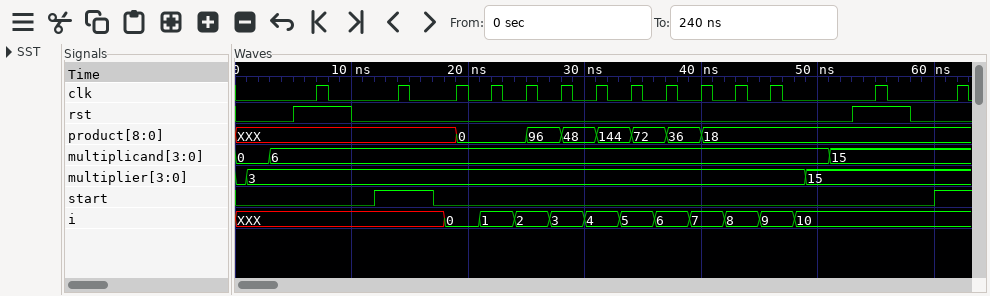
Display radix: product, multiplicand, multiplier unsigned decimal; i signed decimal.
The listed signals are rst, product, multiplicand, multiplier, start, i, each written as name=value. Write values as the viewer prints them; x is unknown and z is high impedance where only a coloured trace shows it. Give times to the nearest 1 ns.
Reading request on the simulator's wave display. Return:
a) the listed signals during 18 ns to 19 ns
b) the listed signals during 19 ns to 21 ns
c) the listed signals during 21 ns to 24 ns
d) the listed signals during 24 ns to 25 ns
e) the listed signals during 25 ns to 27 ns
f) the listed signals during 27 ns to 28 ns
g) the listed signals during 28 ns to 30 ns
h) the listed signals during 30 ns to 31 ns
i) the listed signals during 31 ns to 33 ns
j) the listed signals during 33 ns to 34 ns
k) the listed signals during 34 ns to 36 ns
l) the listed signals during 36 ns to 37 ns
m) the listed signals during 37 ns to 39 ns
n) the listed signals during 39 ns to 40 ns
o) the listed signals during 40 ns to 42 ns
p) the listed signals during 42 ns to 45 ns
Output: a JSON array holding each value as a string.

["rst=0, product=XXX, multiplicand=6, multiplier=3, start=0, i=0", "rst=0, product=0, multiplicand=6, multiplier=3, start=0, i=0", "rst=0, product=0, multiplicand=6, multiplier=3, start=0, i=1", "rst=0, product=0, multiplicand=6, multiplier=3, start=0, i=2", "rst=0, product=96, multiplicand=6, multiplier=3, start=0, i=2", "rst=0, product=96, multiplicand=6, multiplier=3, start=0, i=3", "rst=0, product=48, multiplicand=6, multiplier=3, start=0, i=3", "rst=0, product=48, multiplicand=6, multiplier=3, start=0, i=4", "rst=0, product=144, multiplicand=6, multiplier=3, start=0, i=4", "rst=0, product=144, multiplicand=6, multiplier=3, start=0, i=5", "rst=0, product=72, multiplicand=6, multiplier=3, start=0, i=5", "rst=0, product=72, multiplicand=6, multiplier=3, start=0, i=6", "rst=0, product=36, multiplicand=6, multiplier=3, start=0, i=6", "rst=0, product=36, multiplicand=6, multiplier=3, start=0, i=7", "rst=0, product=18, multiplicand=6, multiplier=3, start=0, i=7", "rst=0, product=18, multiplicand=6, multiplier=3, start=0, i=8"]
